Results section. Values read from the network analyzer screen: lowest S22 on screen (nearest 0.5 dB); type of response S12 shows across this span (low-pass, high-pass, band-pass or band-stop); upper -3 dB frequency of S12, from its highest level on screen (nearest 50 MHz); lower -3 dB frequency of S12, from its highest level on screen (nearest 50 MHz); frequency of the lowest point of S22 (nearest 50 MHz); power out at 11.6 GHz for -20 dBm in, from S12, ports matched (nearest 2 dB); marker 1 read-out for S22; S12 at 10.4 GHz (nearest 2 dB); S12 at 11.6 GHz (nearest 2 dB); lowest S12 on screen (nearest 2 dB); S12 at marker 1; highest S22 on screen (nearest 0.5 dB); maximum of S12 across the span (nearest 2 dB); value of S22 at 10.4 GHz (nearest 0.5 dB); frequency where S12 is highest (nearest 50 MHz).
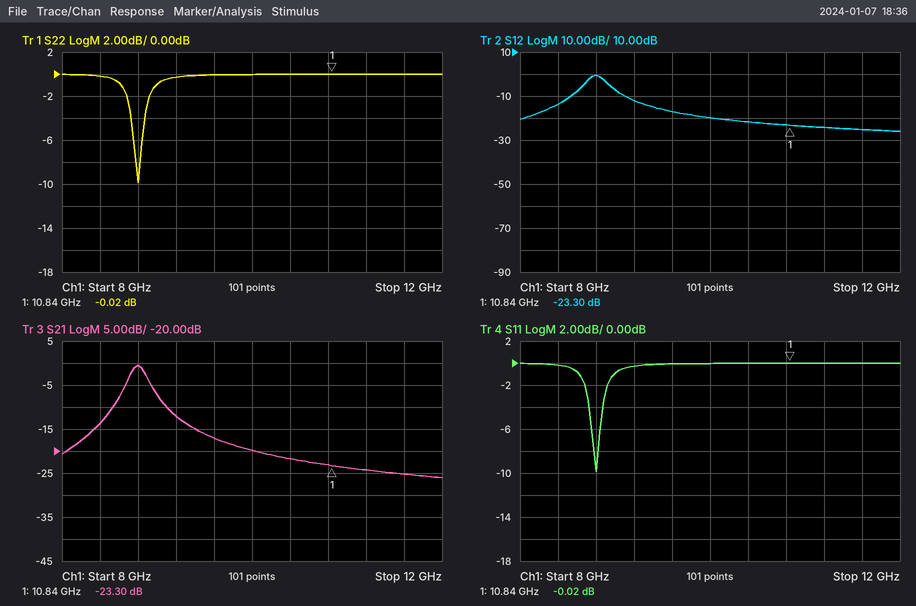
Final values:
-10.0 dB
band-pass
8.90 GHz
8.70 GHz
8.80 GHz
-46 dBm
-0.02 dB
-22 dB
-26 dB
-26 dB
-23.30 dB
0.0 dB
0 dB
0.0 dB
8.80 GHz
